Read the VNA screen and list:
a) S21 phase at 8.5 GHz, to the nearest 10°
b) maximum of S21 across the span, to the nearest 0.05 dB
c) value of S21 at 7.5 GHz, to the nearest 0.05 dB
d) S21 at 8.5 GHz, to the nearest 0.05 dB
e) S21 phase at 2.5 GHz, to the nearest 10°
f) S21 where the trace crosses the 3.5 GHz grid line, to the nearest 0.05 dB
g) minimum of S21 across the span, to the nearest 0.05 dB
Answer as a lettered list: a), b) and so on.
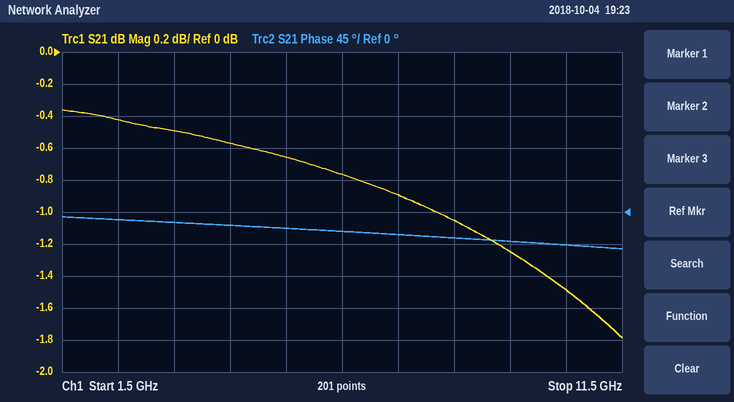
a) -40°
b) -0.35 dB
c) -0.90 dB
d) -1.05 dB
e) -10°
f) -0.50 dB
g) -1.80 dB
